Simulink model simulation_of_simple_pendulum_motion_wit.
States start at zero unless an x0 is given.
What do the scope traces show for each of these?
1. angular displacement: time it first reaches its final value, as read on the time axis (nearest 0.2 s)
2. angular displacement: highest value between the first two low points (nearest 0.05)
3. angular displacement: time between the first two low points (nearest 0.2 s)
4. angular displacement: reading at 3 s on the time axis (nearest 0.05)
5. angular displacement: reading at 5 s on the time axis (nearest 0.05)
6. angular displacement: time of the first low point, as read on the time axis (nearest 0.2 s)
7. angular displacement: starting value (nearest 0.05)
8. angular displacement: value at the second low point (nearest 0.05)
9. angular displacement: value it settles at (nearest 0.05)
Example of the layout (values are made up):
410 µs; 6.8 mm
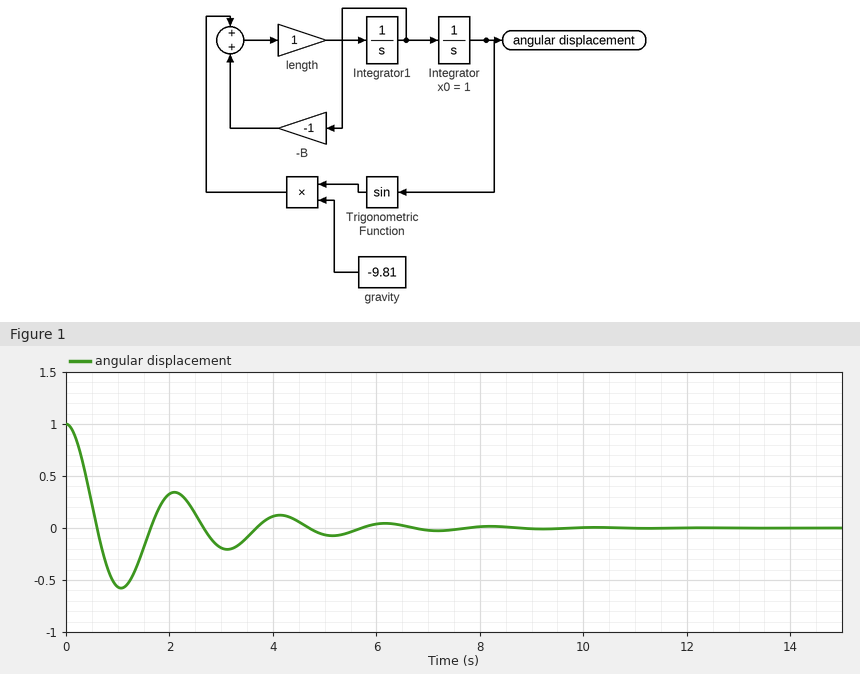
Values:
0.6 s; 0.35; 2.0 s; -0.20; -0.05; 1.0 s; 1.00; -0.20; 0.00
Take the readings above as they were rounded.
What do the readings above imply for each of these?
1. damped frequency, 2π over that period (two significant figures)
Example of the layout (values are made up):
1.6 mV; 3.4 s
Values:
3.1 rad/s
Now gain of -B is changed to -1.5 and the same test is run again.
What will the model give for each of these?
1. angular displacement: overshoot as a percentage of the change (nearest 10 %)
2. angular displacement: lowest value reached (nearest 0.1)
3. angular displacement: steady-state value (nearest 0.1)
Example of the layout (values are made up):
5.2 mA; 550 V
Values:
40 %; -0.4; 0.0
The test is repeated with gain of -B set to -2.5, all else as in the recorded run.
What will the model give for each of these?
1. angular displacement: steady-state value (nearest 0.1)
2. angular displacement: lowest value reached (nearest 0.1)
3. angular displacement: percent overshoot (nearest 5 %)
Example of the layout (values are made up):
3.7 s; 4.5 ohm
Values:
0.0; -0.2; 25 %
